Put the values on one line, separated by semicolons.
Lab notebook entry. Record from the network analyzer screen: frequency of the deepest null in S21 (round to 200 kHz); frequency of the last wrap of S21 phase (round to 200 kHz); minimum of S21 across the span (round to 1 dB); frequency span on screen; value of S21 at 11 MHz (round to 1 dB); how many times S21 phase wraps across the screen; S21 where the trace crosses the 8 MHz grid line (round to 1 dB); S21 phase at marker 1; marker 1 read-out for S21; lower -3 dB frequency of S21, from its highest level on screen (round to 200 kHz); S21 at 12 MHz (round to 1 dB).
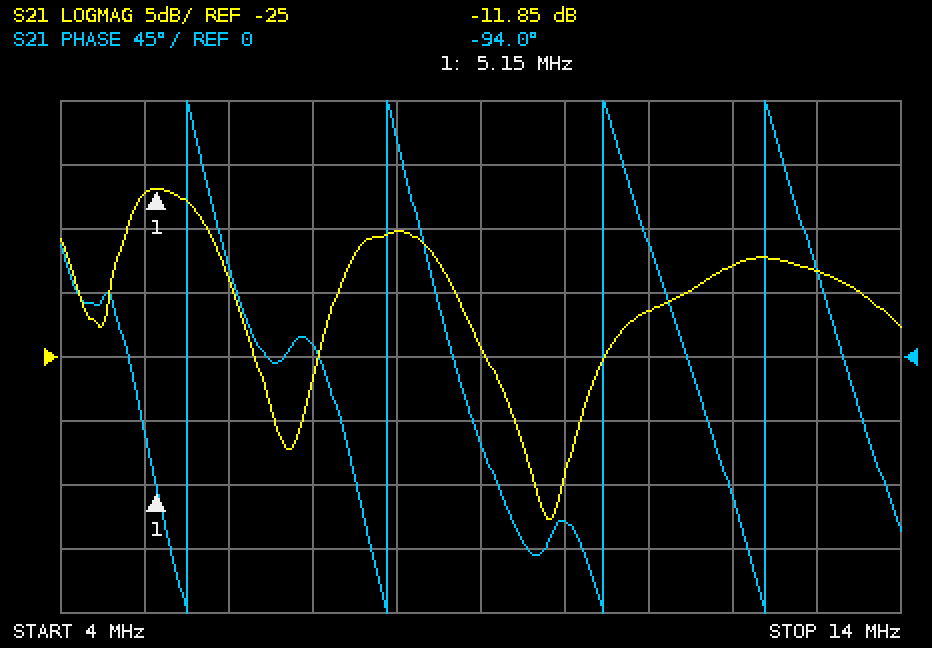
9.8 MHz; 12.4 MHz; -38 dB; 10 MHz; -21 dB; 4; -15 dB; -94.0°; -11.85 dB; 4.8 MHz; -18 dB
